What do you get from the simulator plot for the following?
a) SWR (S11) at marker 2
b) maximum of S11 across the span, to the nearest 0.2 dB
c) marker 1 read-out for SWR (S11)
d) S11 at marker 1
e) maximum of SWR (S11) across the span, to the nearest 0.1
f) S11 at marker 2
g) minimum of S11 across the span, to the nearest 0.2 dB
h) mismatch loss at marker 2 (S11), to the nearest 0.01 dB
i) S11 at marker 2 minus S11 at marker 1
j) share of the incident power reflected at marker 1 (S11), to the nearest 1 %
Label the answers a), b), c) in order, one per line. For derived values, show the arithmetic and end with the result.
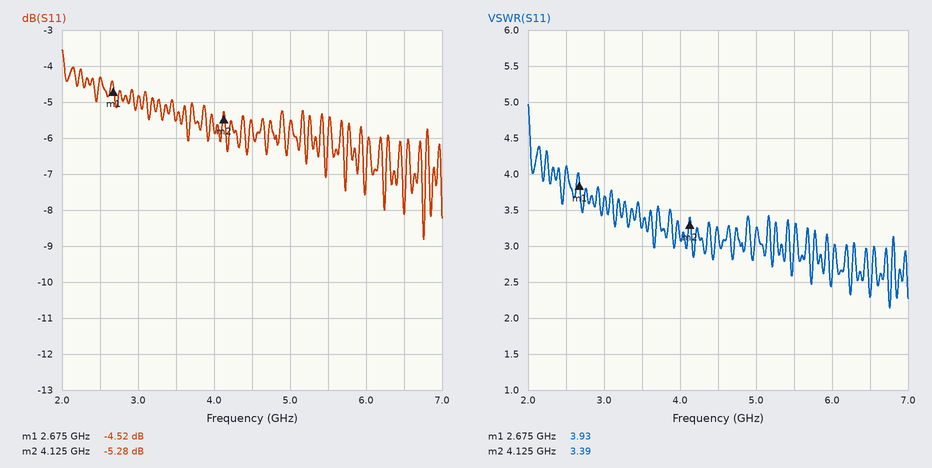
a) 3.39
b) -3.6 dB
c) 3.93
d) -4.52 dB
e) 5.0
f) -5.28 dB
g) -8.8 dB
h) −10 log10(1 − 10^(-5.28/10)) ≈ 1.53 dB
i) -5.28 − (-4.52) = -0.76 dB
j) 10^(-4.52/10) ≈ 35 %
